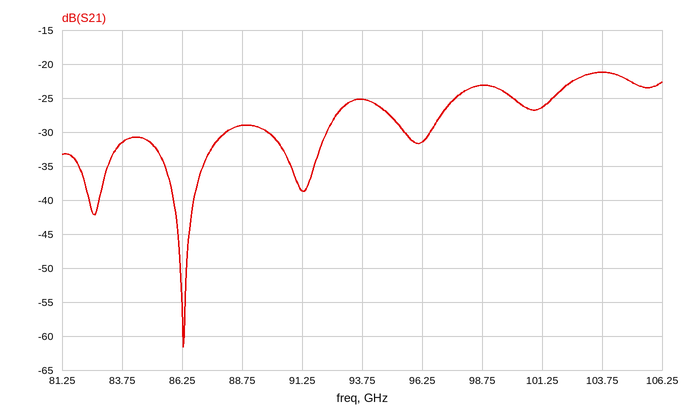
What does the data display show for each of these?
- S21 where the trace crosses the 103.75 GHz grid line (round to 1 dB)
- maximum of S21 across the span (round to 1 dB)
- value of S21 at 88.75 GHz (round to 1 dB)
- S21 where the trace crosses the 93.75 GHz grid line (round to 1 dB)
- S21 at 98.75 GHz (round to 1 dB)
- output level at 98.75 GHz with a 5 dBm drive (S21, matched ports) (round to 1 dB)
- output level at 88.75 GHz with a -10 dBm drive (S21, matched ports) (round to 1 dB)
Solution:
-21 dB
-21 dB
-29 dB
-25 dB
-23 dB
-18 dBm
-39 dBm
